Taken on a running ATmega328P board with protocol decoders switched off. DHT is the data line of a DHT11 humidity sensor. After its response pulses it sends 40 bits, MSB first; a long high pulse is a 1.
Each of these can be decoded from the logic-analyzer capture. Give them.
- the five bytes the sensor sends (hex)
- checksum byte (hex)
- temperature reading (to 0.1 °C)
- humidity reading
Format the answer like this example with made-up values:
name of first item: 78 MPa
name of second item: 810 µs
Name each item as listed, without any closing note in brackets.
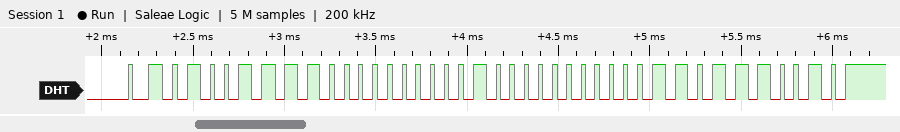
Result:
the five bytes the sensor sends: 4F 00 20 03 72
checksum byte: 0x72
temperature reading: 32.3 °C
humidity reading: 79 %
